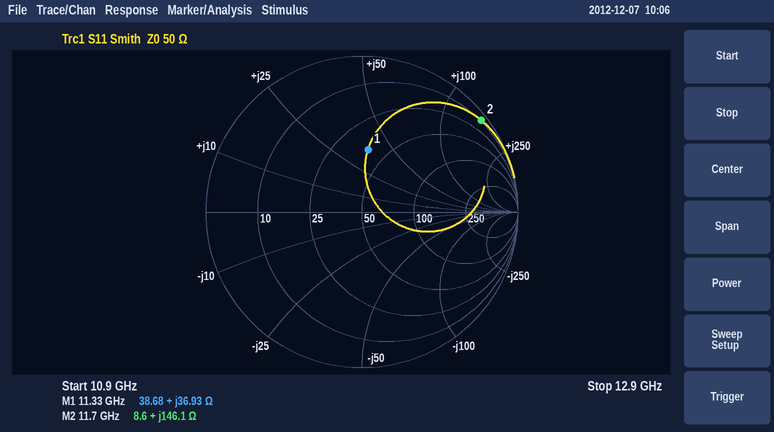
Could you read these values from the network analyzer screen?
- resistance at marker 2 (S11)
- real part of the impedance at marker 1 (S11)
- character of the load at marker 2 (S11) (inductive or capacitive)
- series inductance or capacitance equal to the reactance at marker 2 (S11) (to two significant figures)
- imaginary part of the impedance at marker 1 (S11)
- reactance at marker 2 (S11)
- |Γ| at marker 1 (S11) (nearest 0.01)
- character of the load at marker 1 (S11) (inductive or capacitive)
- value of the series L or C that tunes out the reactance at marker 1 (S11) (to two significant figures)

8.6 Ω
38.68 Ω
inductive
2.0 nH
+36.93 Ω
+146.1 Ω
0.40
inductive
380 fF
